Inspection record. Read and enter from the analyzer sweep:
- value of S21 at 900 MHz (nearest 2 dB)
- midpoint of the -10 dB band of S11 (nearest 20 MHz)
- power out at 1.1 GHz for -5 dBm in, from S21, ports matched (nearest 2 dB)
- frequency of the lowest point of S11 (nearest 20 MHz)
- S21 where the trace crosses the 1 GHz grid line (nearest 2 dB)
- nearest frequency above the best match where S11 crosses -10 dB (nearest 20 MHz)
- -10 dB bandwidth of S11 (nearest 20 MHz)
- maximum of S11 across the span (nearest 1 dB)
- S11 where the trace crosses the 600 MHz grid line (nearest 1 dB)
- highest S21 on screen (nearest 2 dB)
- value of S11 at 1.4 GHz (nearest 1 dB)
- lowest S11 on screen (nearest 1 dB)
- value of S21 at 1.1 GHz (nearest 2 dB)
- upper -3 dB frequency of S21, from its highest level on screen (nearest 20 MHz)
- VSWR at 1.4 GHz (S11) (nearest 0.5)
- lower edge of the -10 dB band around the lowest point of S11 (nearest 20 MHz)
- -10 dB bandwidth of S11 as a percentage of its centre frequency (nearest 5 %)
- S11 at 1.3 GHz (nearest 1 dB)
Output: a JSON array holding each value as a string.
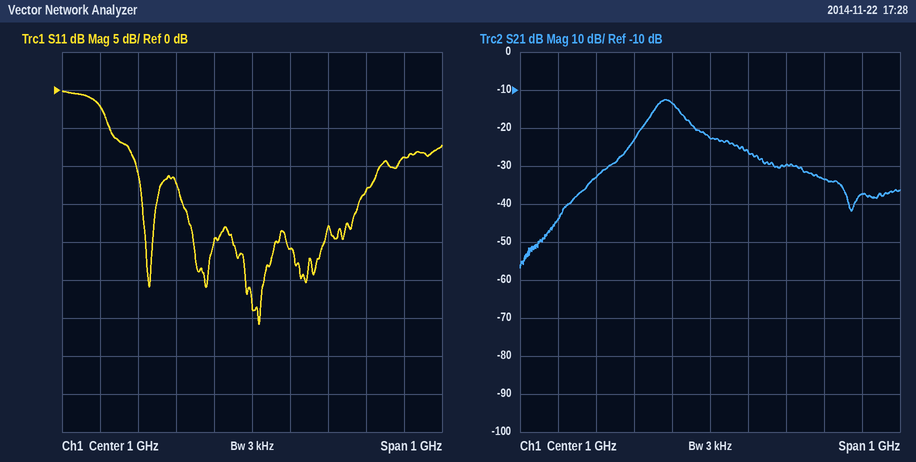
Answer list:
["-14 dB", "1.02 GHz", "-32 dBm", "1.02 GHz", "-22 dB", "1.34 GHz", "640 MHz", "0 dB", "-2 dB", "-12 dB", "-9 dB", "-31 dB", "-26 dB", "920 MHz", "2.0", "700 MHz", "65 %", "-13 dB"]
